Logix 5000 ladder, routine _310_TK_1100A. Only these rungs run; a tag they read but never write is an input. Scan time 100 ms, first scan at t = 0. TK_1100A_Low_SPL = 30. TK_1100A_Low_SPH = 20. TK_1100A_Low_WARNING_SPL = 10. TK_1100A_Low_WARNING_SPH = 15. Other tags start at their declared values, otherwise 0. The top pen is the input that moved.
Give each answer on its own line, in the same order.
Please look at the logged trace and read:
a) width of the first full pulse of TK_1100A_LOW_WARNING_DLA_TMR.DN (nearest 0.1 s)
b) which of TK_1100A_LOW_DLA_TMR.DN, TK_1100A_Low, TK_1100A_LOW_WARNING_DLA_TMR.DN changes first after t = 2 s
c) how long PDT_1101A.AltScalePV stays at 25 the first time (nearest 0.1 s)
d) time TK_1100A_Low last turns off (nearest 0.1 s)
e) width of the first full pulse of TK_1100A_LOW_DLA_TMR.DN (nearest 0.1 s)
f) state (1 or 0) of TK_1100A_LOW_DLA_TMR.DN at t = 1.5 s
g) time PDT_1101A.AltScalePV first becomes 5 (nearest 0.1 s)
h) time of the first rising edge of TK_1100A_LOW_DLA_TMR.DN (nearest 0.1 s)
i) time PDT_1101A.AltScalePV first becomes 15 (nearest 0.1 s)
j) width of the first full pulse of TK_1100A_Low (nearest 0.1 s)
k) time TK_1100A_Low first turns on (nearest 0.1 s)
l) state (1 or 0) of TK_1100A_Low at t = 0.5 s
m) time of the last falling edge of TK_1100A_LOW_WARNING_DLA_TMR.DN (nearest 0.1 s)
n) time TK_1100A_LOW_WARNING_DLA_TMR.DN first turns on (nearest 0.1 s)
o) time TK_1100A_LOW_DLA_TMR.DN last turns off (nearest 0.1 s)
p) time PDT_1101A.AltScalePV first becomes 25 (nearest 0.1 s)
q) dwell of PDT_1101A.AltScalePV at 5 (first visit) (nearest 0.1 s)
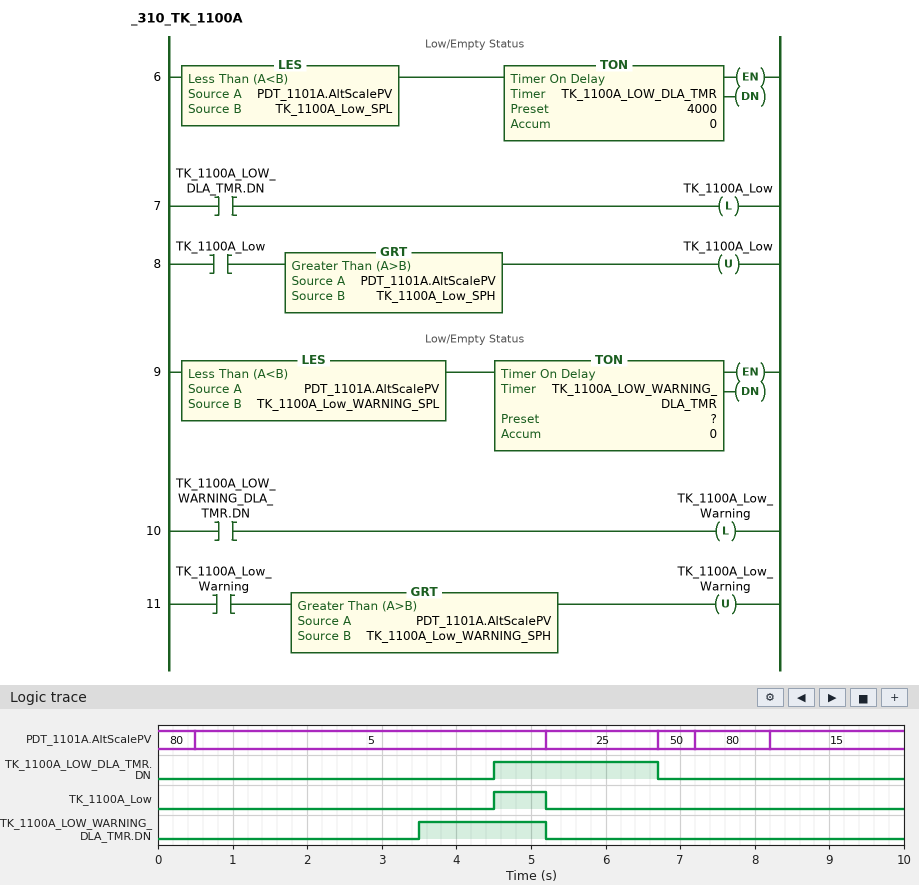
1.7 s
TK_1100A_LOW_WARNING_DLA_TMR.DN
1.5 s
5.2 s
2.2 s
0
0.5 s
4.5 s
8.2 s
0.7 s
4.5 s
0
5.2 s
3.5 s
6.7 s
5.2 s
4.7 s
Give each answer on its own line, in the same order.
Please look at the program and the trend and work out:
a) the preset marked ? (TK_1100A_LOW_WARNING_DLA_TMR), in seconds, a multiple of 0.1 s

3.0 s
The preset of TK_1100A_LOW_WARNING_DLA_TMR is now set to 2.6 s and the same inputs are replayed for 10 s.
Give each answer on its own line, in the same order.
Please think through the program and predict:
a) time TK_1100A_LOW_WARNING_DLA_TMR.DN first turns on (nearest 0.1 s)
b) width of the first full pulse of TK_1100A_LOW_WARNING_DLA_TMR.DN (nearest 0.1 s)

3.1 s
2.1 s
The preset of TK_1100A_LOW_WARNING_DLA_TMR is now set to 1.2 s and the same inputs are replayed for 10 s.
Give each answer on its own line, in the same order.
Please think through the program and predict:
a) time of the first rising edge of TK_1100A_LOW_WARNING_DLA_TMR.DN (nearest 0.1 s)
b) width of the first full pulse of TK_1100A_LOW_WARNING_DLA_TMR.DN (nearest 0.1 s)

1.7 s
3.5 s
